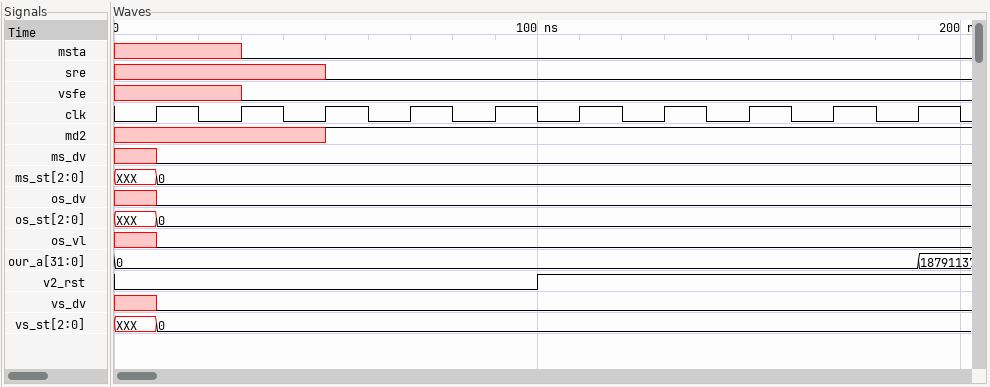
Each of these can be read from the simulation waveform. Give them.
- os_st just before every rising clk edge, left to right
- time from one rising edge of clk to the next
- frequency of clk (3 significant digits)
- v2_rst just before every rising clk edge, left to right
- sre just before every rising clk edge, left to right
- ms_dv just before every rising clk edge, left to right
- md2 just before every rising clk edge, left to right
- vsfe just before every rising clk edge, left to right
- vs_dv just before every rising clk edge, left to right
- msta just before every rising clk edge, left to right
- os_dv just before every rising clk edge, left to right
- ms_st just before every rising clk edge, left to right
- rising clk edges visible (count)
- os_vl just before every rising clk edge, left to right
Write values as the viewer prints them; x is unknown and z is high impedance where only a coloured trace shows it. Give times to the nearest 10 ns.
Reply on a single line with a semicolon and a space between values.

XXX, 0, 0, 0, 0, 0, 0, 0, 0, 0; 20 ns; 50.0 MHz; 0 0 0 0 0 1 1 1 1 1; x x x 0 0 0 0 0 0 0; x 0 0 0 0 0 0 0 0 0; x x x 1 1 1 1 1 1 1; x x 0 0 0 0 0 0 0 0; x 0 0 0 0 0 0 0 0 0; x x 0 0 0 0 0 0 0 0; x 0 0 0 0 0 0 0 0 0; XXX, 0, 0, 0, 0, 0, 0, 0, 0, 0; 10; x 0 0 0 0 0 0 0 0 0
